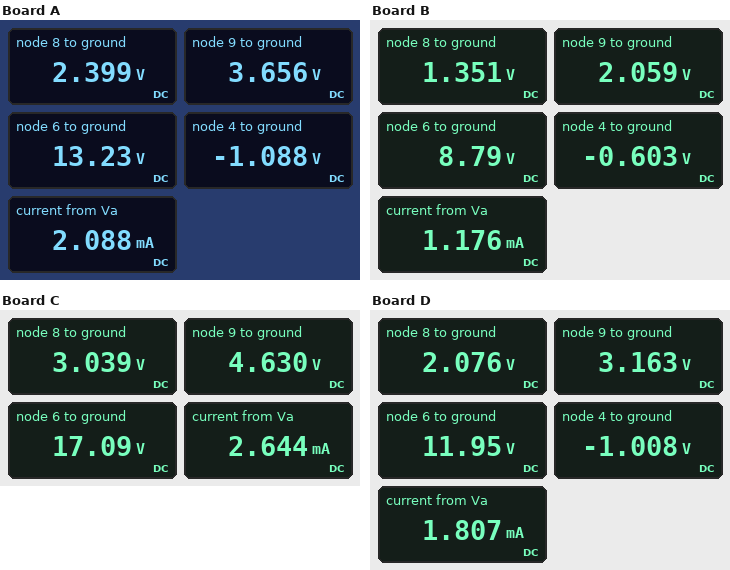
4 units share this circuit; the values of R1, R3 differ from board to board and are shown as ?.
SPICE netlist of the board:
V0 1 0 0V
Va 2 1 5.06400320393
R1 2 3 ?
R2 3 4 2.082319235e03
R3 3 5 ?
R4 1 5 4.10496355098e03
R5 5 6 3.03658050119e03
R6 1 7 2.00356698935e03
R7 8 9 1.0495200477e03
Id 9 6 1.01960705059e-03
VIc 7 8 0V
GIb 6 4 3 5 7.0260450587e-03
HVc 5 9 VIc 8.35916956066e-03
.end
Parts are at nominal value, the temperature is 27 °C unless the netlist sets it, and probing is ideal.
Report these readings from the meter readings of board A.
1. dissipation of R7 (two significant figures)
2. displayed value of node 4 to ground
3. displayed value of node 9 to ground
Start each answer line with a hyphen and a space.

- 1.5 mW
- -1.088 V
- 3.656 V
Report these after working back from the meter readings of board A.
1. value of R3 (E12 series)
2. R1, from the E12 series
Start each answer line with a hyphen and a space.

- 6.8 kΩ
- 820 Ω
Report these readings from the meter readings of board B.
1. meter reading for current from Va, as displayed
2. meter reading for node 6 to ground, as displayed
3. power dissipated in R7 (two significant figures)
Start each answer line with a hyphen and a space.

- 1.176 mA
- 8.79 V
- 480 µW
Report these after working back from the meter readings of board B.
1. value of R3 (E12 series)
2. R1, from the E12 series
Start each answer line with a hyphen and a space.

- 8.2 kΩ
- 2.7 kΩ
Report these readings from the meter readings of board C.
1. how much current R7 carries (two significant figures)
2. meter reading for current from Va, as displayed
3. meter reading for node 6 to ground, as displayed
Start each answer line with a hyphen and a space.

- 1.5 mA
- 2.644 mA
- 17.09 V
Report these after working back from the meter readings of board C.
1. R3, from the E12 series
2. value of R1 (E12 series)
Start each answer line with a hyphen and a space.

- 1 kΩ
- 330 Ω
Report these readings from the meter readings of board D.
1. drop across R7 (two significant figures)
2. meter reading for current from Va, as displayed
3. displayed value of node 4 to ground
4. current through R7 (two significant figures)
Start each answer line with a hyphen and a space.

- 1.1 V
- 1.807 mA
- -1.008 V
- 1.0 mA
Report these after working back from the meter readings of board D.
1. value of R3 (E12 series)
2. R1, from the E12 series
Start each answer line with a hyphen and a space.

- 3.9 kΩ
- 1.2 kΩ
